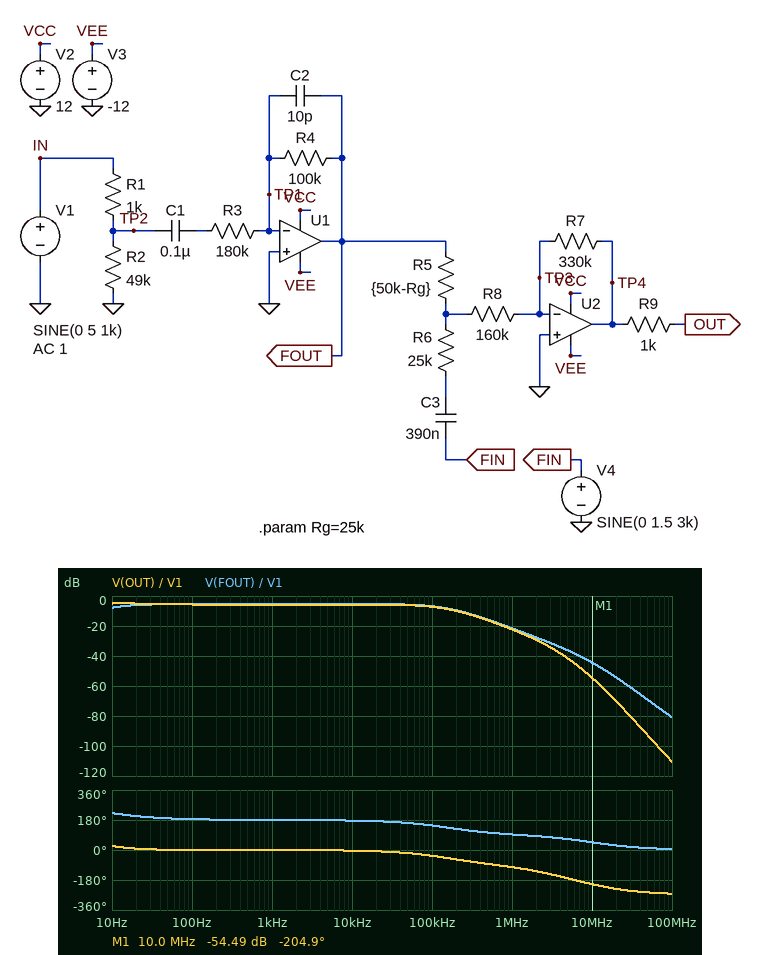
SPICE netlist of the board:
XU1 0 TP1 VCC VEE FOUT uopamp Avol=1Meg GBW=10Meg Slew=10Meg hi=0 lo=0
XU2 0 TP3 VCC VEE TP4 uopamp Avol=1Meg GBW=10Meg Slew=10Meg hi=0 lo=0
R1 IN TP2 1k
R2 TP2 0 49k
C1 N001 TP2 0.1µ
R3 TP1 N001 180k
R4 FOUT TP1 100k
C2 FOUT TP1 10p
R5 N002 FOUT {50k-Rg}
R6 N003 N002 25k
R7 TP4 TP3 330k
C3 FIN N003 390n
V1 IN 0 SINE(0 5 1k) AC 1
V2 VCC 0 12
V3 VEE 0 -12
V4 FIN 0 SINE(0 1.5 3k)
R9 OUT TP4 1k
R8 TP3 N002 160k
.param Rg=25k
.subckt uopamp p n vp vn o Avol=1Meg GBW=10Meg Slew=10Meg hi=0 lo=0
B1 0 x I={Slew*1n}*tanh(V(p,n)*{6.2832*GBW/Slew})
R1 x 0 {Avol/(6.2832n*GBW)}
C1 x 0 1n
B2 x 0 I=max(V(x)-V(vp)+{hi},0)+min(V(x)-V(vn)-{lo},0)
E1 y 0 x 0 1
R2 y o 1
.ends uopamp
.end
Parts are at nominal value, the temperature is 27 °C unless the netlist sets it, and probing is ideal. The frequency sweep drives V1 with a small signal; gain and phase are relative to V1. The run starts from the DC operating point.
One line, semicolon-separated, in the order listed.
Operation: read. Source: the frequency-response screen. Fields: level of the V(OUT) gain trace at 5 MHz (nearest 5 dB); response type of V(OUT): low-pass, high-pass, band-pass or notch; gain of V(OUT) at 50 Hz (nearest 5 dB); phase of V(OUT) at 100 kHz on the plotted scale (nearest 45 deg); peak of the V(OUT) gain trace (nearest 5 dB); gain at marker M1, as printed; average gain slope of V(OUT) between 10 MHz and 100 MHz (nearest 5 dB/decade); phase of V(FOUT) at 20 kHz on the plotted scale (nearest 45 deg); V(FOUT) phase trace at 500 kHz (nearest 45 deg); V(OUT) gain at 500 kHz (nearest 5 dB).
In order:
-40 dB; low-pass; -5 dB; -45 deg; -5 dB; -54.49 dB; -55 dB/decade; 180 deg; 90 deg; -15 dB
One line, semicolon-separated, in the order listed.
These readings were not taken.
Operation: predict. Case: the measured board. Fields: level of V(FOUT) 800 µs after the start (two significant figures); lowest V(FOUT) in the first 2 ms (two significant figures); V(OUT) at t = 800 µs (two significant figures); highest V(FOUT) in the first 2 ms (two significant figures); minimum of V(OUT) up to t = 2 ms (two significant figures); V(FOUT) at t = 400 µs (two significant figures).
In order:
2.6 V; -2.7 V; -3.3 V; 2.7 V; -4.0 V; -1.6 V
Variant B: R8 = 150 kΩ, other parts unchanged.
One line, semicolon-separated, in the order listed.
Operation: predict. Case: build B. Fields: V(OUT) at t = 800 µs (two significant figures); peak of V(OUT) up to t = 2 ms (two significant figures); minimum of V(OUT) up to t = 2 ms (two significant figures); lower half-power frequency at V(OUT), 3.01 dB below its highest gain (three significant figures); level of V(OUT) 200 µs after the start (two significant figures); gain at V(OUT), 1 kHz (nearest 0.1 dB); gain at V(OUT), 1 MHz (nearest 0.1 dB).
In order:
-3.5 V; 4.3 V; -4.3 V; 4.48 Hz; 3.5 V; -5.2 dB; -21.8 dB
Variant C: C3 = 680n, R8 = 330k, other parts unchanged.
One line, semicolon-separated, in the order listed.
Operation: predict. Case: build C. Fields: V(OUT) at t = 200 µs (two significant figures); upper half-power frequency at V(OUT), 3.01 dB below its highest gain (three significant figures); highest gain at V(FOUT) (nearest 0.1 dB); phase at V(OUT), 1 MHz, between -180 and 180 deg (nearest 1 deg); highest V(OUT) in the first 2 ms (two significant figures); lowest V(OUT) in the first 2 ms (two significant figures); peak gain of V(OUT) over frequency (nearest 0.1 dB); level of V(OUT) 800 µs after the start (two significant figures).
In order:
1.7 V; 158 kHz; -5.3 dB; -98 deg; 2.0 V; -2.0 V; -11.7 dB; -1.7 V
